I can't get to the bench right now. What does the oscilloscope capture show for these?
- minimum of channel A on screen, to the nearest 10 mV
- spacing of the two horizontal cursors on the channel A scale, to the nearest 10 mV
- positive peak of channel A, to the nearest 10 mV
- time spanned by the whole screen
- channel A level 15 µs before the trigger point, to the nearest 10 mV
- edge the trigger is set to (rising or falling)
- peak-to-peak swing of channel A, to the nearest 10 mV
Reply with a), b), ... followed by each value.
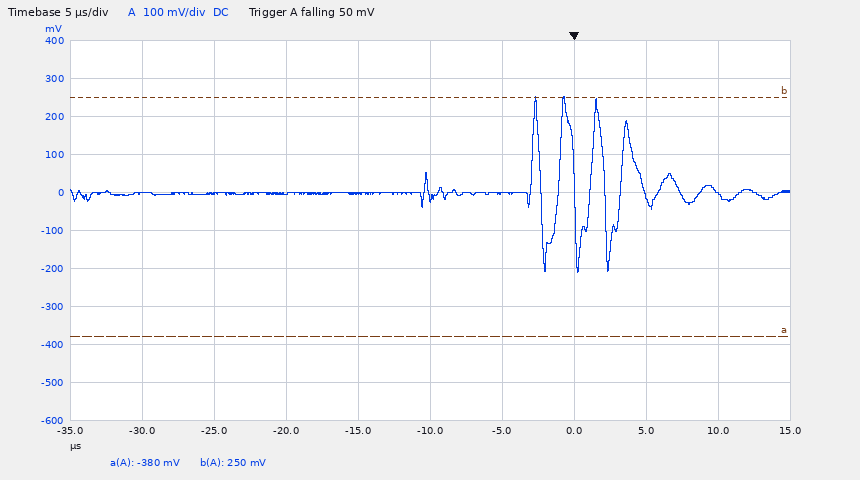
a) -210 mV
b) 630 mV
c) 250 mV
d) 50 µs
e) 0 mV
f) falling
g) 460 mV
